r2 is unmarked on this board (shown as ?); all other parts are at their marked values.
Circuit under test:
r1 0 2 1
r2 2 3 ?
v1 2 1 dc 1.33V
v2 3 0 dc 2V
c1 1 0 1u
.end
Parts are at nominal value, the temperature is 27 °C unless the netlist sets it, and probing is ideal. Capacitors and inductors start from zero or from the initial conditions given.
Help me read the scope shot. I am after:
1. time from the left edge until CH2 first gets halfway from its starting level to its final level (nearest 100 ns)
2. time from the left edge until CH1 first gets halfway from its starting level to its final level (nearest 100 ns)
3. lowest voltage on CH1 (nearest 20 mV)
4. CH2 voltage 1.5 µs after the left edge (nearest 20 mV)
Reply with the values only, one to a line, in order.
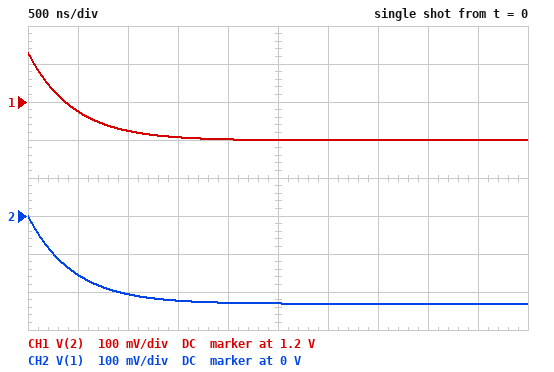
300 ns
300 ns
1.10 V
-220 mV
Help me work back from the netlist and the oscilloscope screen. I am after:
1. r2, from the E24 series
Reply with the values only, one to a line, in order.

0.82 Ω
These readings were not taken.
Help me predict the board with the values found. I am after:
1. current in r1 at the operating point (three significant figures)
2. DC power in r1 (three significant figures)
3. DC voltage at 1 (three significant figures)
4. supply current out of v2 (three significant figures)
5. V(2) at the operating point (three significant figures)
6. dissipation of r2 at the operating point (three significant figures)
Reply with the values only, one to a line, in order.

1.10 A
1.21 W
-231 mV
1.10 A
1.10 V
990 mW
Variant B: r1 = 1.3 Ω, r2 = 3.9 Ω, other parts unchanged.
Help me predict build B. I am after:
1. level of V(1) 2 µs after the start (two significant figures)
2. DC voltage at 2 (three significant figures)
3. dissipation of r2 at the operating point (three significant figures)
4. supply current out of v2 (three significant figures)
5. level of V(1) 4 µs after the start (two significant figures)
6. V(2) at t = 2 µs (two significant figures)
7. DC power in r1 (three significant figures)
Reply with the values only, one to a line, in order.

-720 mV
500 mV
577 mW
385 mA
-820 mV
610 mV
192 mW
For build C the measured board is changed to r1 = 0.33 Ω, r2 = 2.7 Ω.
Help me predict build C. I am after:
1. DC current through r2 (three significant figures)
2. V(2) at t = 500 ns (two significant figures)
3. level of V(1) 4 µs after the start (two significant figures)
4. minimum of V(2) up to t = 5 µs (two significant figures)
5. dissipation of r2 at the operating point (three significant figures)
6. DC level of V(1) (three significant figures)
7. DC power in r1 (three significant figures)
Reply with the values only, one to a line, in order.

660 mA
420 mV
-1.1 V
220 mV
1.18 W
-1.11 V
144 mW
